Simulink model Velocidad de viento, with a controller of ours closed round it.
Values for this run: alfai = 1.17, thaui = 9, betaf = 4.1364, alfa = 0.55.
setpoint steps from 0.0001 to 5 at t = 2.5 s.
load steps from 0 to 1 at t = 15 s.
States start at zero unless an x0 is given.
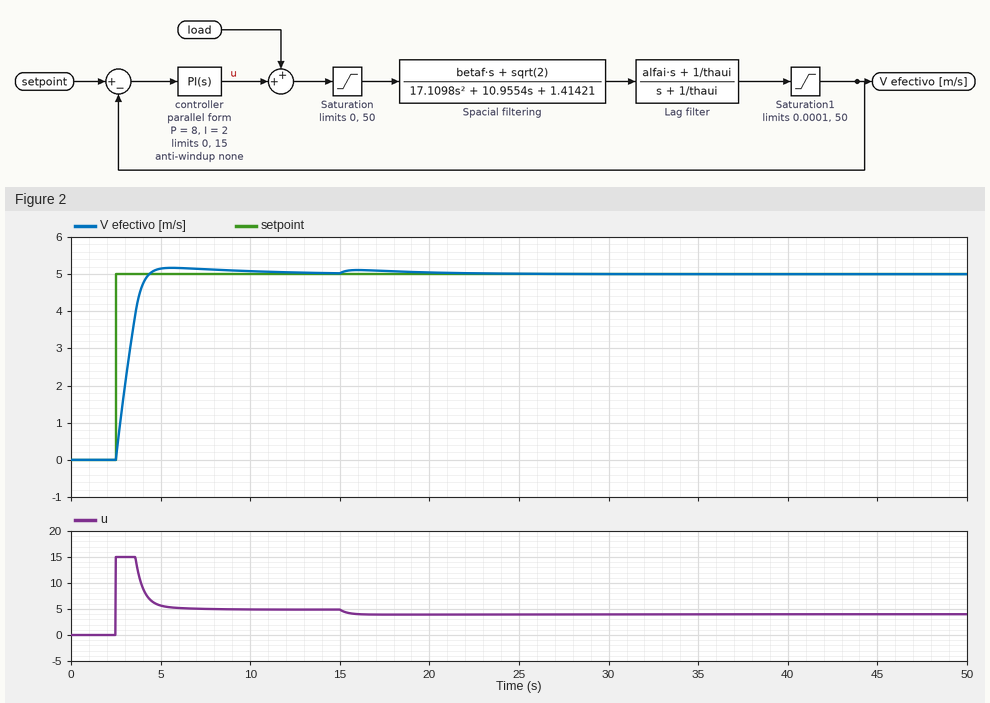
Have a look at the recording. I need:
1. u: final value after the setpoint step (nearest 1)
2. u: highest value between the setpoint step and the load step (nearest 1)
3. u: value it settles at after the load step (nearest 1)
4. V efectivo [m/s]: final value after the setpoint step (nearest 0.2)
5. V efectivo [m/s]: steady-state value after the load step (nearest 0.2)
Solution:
5
15
4
5.0
5.0
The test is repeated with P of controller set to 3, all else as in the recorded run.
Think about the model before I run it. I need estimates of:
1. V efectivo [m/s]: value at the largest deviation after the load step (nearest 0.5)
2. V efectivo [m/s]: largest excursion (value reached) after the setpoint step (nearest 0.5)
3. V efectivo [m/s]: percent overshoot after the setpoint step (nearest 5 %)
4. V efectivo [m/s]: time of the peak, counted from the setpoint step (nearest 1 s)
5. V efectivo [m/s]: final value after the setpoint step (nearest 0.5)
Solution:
5.0
5.5
10 %
4 s
5.0
